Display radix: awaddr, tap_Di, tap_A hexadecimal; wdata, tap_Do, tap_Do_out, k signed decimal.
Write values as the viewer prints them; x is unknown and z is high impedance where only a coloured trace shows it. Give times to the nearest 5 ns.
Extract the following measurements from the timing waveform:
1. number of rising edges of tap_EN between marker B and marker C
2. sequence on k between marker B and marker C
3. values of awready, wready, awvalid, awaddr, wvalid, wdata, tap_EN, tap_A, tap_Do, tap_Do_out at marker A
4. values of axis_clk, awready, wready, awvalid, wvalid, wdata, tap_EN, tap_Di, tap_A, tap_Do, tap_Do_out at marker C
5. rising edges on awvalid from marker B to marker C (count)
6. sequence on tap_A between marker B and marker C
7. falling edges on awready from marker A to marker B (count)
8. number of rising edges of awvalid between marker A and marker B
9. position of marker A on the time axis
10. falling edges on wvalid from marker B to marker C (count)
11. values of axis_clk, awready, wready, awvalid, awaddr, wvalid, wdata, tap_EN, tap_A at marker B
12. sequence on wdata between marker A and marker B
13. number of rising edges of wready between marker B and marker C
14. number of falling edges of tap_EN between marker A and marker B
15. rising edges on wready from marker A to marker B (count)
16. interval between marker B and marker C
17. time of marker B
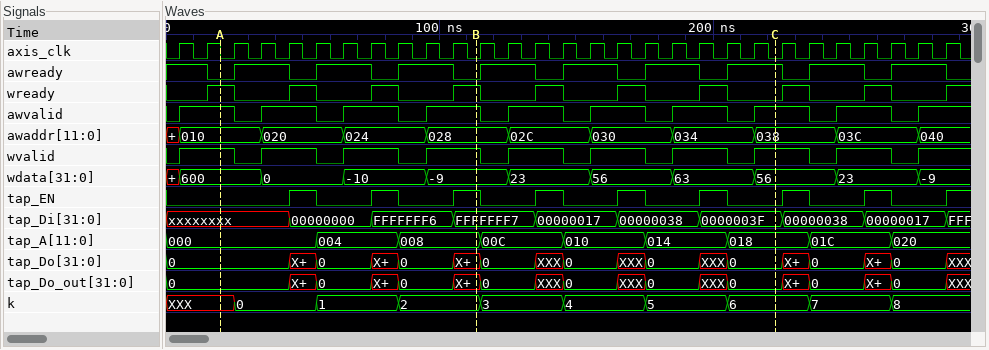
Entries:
3
2, 3, 4, 5, 6
awready=0, wready=1, awvalid=1, awaddr=010, wvalid=1, wdata=600, tap_EN=0, tap_A=000, tap_Do=0, tap_Do_out=0
axis_clk=0, awready=1, wready=0, awvalid=1, wvalid=1, wdata=56, tap_EN=0, tap_Di=0000003F, tap_A=018, tap_Do=0, tap_Do_out=0
4
008, 00C, 010, 014, 018
3
3
20 ns
4
axis_clk=0, awready=0, wready=1, awvalid=1, awaddr=028, wvalid=1, wdata=-9, tap_EN=1, tap_A=008
600, 0, -10, -9
3
2
3
110 ns
115 ns
